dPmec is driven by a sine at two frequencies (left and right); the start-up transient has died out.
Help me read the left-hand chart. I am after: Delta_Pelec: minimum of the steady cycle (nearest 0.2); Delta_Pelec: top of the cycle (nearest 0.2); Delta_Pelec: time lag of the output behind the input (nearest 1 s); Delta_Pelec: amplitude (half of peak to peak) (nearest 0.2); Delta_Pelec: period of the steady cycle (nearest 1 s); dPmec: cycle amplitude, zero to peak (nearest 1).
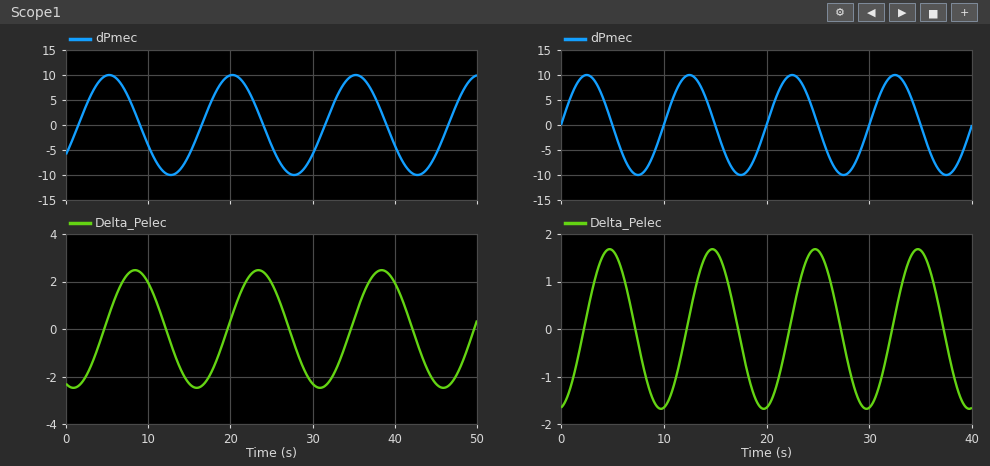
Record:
-2.4
2.4
3 s
2.4
15 s
10
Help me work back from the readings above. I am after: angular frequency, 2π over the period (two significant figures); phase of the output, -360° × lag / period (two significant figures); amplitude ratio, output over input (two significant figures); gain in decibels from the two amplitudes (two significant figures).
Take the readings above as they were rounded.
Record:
0.42 rad/s
-72°
0.24
-12 dB
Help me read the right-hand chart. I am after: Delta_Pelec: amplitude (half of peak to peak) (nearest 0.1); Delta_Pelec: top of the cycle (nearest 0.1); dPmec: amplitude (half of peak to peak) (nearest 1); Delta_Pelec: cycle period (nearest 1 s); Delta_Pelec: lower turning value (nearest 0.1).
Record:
1.7
1.7
10
10 s
-1.7
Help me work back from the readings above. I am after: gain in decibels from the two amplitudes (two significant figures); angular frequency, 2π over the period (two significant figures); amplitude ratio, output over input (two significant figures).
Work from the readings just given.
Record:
-15 dB
0.63 rad/s
0.17
